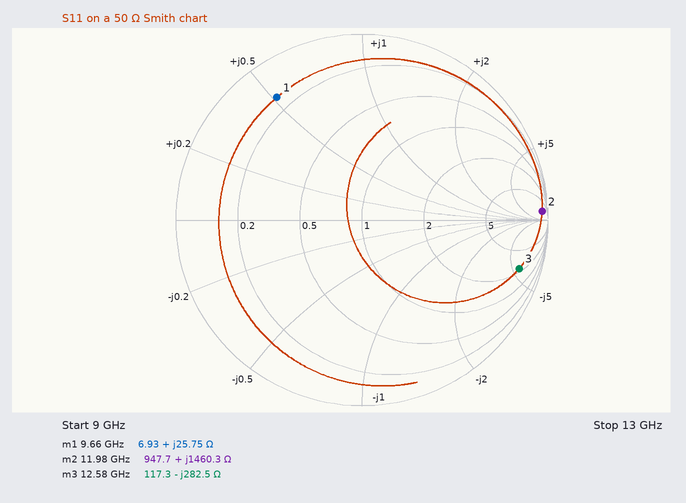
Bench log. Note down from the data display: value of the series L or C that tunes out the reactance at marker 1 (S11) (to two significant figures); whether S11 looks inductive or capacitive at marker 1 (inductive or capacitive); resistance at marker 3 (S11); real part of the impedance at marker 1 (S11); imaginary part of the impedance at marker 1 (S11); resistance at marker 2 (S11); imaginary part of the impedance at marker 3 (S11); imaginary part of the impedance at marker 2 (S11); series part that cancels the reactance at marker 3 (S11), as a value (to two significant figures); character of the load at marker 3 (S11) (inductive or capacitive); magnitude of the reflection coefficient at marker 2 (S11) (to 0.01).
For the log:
640 fF
inductive
117.3 Ω
6.93 Ω
+25.75 Ω
947.7 Ω
-282.5 Ω
+1460.3 Ω
3.6 nH
capacitive
0.97
